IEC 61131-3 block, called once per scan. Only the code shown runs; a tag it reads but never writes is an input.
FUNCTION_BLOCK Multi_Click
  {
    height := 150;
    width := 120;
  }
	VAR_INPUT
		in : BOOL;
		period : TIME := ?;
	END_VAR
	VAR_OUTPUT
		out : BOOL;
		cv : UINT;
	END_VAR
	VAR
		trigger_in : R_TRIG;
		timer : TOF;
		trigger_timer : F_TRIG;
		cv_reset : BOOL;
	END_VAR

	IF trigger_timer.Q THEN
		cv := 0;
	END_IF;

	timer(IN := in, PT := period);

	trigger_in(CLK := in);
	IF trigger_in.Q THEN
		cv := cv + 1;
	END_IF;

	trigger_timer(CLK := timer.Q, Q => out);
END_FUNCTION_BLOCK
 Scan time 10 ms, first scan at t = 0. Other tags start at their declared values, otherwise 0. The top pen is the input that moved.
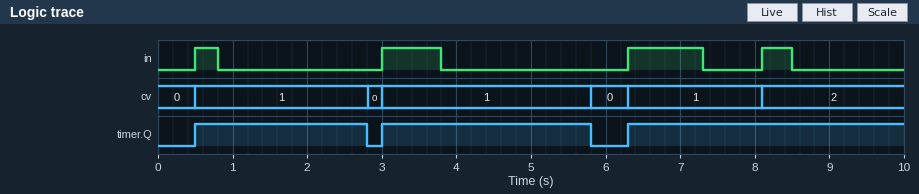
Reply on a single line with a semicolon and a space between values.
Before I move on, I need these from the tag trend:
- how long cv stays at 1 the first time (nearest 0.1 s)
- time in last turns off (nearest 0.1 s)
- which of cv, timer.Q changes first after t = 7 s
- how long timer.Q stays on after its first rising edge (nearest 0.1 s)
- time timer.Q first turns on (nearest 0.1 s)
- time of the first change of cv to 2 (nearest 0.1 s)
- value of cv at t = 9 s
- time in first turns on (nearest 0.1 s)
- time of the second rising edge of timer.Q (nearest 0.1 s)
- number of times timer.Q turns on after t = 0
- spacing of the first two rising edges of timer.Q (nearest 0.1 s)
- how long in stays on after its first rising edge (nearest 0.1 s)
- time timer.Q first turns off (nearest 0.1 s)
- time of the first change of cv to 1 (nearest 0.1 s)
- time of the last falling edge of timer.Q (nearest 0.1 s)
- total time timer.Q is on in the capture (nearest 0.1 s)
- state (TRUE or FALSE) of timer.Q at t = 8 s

2.3 s; 8.5 s; cv; 2.3 s; 0.5 s; 8.1 s; 2; 0.5 s; 3.0 s; 3; 2.5 s; 0.3 s; 2.8 s; 0.5 s; 5.8 s; 8.8 s; TRUE
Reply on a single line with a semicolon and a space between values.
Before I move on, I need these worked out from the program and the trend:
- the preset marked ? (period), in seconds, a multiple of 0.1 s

2.0 s
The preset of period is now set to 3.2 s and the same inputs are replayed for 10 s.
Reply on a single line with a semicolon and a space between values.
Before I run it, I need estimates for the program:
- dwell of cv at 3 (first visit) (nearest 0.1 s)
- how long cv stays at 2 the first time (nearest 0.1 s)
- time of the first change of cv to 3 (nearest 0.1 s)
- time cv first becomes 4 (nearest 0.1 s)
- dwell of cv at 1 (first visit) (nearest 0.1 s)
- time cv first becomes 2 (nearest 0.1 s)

1.8 s; 3.3 s; 6.3 s; 8.1 s; 2.5 s; 3.0 s
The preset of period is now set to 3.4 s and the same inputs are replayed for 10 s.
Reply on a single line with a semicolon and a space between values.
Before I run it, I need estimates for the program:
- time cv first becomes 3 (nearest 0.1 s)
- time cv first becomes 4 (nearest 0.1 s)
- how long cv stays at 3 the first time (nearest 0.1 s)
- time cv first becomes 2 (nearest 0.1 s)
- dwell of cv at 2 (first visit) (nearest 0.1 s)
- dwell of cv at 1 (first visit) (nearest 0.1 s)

6.3 s; 8.1 s; 1.8 s; 3.0 s; 3.3 s; 2.5 s
